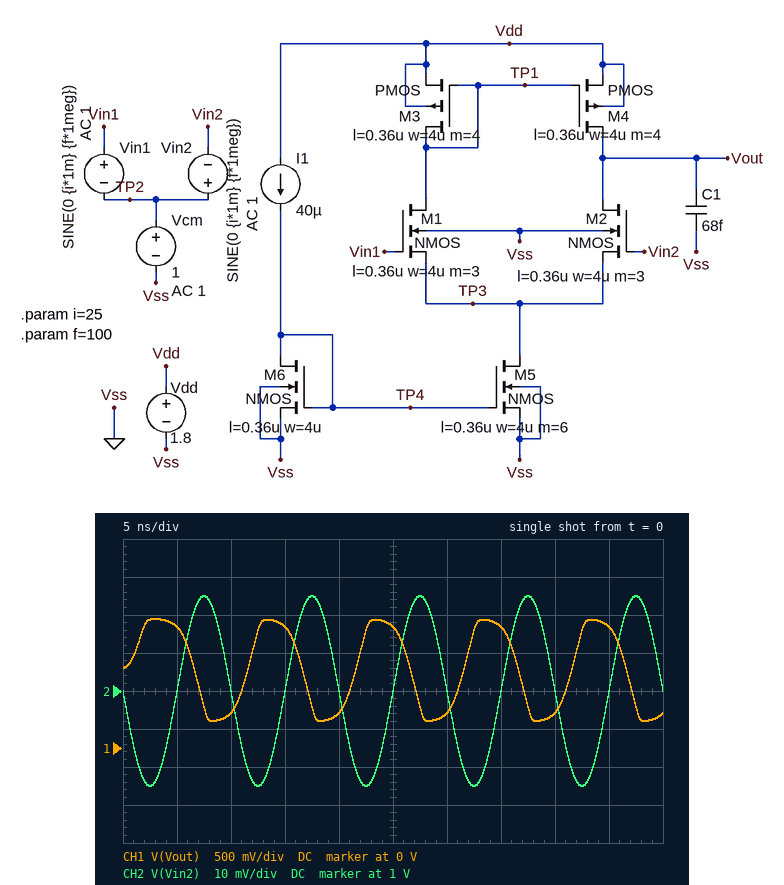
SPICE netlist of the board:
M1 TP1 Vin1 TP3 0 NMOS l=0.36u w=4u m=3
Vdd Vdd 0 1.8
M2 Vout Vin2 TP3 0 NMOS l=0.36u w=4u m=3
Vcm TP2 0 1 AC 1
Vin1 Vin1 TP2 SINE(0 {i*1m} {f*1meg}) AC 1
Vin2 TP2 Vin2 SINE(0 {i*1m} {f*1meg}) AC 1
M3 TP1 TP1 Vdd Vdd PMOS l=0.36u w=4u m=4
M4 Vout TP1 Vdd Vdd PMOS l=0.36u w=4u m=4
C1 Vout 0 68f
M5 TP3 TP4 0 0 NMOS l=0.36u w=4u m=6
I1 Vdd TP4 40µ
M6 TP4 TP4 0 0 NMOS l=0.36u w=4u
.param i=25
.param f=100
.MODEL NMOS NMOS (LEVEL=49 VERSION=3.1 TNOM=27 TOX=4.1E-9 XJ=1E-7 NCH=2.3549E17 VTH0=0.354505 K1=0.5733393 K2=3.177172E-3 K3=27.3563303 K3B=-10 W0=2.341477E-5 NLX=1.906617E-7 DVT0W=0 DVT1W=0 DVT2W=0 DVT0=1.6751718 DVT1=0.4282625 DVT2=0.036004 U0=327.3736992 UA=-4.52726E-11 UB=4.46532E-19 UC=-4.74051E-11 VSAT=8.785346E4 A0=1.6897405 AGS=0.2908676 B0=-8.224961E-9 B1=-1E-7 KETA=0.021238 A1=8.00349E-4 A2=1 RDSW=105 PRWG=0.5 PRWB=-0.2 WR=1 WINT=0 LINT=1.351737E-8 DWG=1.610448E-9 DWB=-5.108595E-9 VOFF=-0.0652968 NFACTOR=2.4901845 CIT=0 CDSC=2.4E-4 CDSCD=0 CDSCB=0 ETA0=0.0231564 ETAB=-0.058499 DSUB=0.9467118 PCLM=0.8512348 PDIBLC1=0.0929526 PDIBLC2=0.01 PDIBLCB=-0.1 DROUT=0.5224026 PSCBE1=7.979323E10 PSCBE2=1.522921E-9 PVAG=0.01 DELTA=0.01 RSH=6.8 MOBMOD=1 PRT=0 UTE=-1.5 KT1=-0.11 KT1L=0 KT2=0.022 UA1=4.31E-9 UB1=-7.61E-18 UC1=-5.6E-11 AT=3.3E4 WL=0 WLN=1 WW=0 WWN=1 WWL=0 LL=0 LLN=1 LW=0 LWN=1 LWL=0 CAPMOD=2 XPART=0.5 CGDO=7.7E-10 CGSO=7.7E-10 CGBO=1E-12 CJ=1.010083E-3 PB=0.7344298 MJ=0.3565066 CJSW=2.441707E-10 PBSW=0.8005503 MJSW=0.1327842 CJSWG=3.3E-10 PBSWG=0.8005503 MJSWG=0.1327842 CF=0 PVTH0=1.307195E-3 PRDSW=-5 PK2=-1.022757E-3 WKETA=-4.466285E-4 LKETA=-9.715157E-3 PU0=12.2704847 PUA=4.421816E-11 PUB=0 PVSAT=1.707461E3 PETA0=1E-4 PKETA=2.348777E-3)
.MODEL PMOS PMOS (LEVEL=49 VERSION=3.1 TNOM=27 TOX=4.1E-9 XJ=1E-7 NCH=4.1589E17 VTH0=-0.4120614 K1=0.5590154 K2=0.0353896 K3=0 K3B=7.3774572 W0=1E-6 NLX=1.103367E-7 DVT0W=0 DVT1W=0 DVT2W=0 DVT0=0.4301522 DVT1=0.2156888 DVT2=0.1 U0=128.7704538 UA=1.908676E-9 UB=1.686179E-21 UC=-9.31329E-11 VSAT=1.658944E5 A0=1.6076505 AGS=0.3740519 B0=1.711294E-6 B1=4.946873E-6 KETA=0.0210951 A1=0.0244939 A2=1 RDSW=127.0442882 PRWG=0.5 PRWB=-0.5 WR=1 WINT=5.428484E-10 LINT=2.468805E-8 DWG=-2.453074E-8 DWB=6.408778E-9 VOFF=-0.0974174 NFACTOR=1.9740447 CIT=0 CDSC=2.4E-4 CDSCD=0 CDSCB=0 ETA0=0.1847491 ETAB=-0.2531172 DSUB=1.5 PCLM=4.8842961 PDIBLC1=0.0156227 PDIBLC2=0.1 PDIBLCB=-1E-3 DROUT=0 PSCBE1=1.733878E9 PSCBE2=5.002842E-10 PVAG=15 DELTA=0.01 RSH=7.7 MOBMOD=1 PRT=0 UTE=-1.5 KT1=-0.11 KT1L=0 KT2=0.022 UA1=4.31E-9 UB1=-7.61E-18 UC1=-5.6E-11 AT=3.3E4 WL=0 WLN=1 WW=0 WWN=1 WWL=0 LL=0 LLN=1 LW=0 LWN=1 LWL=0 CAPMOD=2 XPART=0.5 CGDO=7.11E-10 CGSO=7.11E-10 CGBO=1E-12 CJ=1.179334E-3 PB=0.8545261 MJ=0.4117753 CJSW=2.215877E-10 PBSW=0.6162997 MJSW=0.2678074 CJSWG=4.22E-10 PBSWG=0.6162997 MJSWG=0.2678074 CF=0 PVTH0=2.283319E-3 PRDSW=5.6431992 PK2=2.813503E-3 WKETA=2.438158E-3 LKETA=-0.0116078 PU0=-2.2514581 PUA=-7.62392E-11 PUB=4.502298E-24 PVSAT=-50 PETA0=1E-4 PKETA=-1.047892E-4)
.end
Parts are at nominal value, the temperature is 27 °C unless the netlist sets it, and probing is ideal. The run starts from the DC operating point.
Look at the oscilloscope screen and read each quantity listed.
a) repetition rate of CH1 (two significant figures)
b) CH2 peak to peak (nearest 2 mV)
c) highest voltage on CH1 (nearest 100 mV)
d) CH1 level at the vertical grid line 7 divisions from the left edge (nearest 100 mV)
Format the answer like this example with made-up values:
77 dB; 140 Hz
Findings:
100 MHz; 50 mV; 1.7 V; 1.6 V
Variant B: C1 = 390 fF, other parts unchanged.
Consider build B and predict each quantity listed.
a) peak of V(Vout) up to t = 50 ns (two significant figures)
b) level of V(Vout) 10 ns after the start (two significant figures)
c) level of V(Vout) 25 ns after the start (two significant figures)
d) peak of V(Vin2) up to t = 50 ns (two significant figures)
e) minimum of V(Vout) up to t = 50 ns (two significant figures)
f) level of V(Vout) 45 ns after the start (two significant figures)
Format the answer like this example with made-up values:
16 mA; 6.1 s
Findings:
1.5 V; 950 mV; 1.4 V; 1.0 V; 820 mV; 1.3 V
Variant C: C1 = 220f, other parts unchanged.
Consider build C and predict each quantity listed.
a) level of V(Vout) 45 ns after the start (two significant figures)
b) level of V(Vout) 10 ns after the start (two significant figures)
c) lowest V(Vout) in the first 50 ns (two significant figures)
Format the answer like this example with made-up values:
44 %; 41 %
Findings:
1.5 V; 720 mV; 640 mV
